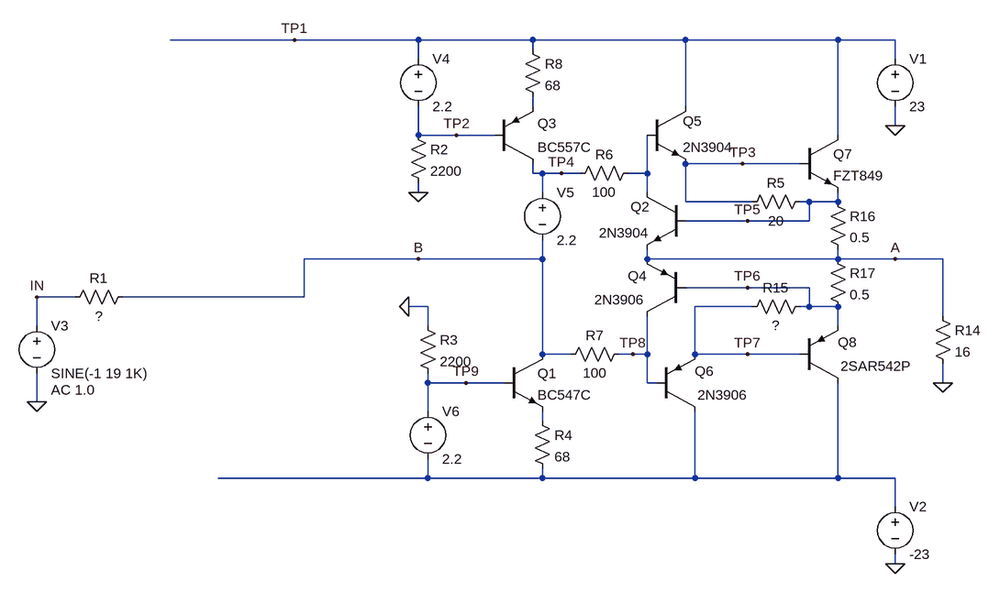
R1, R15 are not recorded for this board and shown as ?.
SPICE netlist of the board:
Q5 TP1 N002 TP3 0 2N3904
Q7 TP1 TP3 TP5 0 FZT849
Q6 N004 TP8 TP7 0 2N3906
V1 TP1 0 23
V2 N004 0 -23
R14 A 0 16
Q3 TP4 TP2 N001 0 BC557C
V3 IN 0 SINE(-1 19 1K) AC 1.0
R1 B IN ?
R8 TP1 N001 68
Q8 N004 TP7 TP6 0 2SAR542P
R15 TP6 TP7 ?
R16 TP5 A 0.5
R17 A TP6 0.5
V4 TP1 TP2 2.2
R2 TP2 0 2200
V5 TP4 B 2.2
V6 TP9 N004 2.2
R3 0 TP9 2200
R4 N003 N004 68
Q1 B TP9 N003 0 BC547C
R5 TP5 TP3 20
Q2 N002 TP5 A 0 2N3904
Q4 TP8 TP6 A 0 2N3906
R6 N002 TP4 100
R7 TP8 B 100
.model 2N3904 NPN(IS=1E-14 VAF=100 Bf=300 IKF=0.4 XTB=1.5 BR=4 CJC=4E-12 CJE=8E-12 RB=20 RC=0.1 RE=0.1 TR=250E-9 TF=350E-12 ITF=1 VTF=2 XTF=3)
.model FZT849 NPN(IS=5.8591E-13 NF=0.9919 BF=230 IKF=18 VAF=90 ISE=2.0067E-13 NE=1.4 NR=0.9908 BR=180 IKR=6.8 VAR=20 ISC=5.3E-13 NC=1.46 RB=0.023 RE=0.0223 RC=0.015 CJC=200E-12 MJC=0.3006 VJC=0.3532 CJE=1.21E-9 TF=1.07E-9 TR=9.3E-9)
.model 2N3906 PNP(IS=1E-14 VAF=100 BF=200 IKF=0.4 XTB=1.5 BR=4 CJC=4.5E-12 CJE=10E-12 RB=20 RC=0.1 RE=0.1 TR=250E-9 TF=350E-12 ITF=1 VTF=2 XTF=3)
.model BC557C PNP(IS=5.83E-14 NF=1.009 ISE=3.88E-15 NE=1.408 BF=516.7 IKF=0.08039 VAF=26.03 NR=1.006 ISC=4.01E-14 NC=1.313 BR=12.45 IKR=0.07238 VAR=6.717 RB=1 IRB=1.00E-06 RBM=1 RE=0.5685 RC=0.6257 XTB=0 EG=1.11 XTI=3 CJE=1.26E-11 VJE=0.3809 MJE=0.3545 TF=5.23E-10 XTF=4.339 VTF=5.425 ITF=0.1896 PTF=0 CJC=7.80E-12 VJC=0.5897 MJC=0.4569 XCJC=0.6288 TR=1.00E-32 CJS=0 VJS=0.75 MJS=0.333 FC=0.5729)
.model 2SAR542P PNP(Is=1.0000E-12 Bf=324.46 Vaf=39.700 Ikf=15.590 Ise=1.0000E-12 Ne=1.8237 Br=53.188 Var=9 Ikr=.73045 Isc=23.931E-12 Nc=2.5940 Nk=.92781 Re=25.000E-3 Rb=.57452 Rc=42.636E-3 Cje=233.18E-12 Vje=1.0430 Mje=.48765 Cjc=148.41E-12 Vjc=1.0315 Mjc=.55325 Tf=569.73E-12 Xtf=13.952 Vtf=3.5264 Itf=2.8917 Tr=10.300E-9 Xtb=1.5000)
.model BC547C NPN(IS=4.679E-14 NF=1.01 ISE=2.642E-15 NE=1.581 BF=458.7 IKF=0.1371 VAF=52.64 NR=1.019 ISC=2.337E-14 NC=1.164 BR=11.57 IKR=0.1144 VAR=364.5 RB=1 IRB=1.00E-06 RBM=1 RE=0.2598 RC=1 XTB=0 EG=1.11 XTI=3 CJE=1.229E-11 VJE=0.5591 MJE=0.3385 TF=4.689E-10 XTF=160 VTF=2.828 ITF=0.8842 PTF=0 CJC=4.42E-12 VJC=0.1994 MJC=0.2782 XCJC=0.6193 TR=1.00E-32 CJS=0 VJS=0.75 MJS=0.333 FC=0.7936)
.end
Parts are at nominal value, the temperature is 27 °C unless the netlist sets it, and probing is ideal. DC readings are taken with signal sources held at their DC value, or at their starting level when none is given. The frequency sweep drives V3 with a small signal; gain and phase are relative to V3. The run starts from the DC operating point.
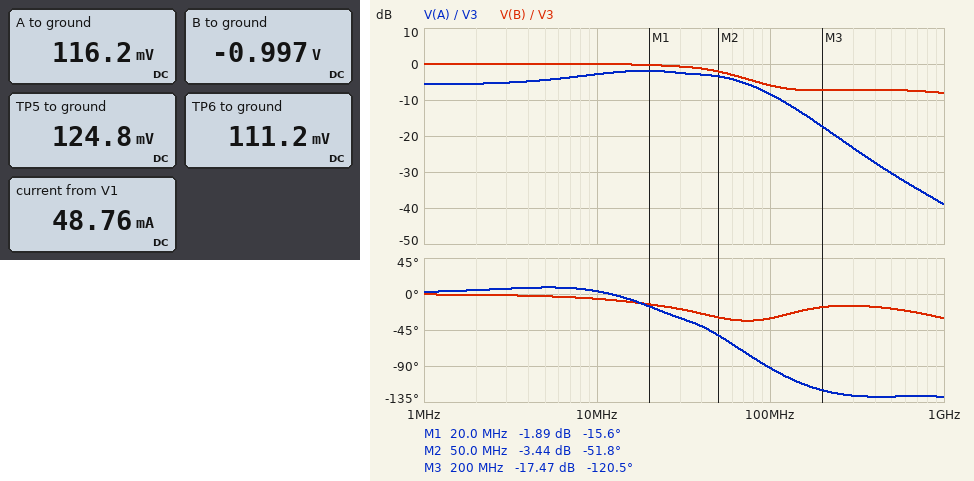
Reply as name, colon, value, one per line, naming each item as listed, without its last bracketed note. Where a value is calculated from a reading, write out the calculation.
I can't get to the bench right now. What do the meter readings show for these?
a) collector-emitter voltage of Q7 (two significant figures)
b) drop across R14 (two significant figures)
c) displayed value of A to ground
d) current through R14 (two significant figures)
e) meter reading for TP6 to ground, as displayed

collector-emitter voltage of Q7: 23 V - 124.8 mV = 23 V
drop across R14: 116.2 mV = 120 mV
displayed value of A to ground: 116.2 mV
current through R14: (116.2 mV) / 16 Ω = 7.3 mA
meter reading for TP6 to ground, as displayed: 111.2 mV
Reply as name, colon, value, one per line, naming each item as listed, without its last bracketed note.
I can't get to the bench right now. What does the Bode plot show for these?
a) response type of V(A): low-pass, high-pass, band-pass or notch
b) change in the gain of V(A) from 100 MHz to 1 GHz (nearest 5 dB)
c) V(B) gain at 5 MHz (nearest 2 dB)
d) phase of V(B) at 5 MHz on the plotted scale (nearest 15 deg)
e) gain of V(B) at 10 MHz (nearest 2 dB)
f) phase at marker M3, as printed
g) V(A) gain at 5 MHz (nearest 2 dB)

response type of V(A): low-pass, high-pass, band-pass or notch: low-pass
change in the gain of V(A) from 100 MHz to 1 GHz: -30 dB
V(B) gain at 5 MHz: 0 dB
phase of V(B) at 5 MHz on the plotted scale: 0 deg
gain of V(B) at 10 MHz: 0 dB
phase at marker M3, as printed: -120.5 deg
V(A) gain at 5 MHz: -4 dB
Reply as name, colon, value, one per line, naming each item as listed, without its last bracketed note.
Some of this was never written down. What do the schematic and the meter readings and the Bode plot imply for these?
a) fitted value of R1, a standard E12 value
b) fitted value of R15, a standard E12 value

fitted value of R1, a standard E12 value: 68 Ω
fitted value of R15, a standard E12 value: 39 Ω
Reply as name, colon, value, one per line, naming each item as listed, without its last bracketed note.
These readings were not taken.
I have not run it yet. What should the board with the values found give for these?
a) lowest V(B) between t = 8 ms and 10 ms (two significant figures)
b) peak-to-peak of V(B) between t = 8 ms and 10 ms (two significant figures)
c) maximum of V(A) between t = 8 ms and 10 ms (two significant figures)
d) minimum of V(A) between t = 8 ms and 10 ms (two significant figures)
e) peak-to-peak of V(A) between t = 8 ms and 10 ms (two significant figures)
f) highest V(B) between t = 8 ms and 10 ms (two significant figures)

lowest V(B) between t = 8 ms and 10 ms: -20 V
peak-to-peak of V(B) between t = 8 ms and 10 ms: 38 V
maximum of V(A) between t = 8 ms and 10 ms: 18 V
minimum of V(A) between t = 8 ms and 10 ms: -18 V
peak-to-peak of V(A) between t = 8 ms and 10 ms: 36 V
highest V(B) between t = 8 ms and 10 ms: 18 V
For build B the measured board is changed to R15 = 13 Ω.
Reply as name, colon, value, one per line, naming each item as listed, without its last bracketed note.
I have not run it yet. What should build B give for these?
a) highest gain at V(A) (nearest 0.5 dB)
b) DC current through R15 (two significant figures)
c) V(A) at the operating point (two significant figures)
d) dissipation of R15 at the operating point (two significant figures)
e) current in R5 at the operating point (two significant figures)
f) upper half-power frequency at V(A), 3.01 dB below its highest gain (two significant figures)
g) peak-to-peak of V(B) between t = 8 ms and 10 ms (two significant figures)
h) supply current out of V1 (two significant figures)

highest gain at V(A): -1.5 dB
DC current through R15: 20 mA
V(A) at the operating point: 21 mV
dissipation of R15 at the operating point: 5.4 mW
current in R5 at the operating point: 22 mA
upper half-power frequency at V(A), 3.01 dB below its highest gain: 66 MHz
peak-to-peak of V(B) between t = 8 ms and 10 ms: 38 V
supply current out of V1: 53 mA
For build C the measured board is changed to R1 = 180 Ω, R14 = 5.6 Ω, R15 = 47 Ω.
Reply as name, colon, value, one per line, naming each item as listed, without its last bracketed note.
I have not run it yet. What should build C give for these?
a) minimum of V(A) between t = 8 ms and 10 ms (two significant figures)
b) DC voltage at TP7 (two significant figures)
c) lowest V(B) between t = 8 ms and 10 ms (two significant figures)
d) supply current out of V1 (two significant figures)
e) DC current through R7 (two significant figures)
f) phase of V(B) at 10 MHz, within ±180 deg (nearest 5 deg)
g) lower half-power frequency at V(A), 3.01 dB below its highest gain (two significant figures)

minimum of V(A) between t = 8 ms and 10 ms: -8.5 V
DC voltage at TP7: -290 mV
lowest V(B) between t = 8 ms and 10 ms: -13 V
supply current out of V1: 51 mA
DC current through R7: 31 µA
phase of V(B) at 10 MHz, within ±180 deg: -25 deg
lower half-power frequency at V(A), 3.01 dB below its highest gain: 5.0 MHz
